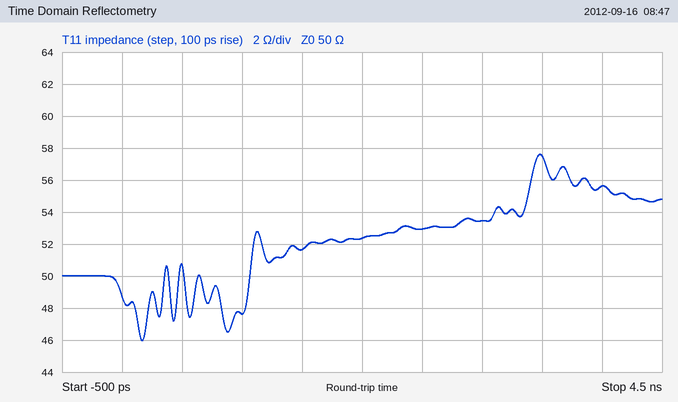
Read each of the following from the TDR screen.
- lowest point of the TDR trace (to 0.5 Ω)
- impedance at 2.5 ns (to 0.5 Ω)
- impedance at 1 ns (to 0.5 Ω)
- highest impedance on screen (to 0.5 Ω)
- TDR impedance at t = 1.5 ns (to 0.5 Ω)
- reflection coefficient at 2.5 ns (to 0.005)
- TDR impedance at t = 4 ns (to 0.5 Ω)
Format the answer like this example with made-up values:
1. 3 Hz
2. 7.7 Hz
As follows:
1. 46.0 Ω
2. 53.0 Ω
3. 47.5 Ω
4. 57.5 Ω
5. 51.5 Ω
6. +0.030
7. 55.5 Ω
